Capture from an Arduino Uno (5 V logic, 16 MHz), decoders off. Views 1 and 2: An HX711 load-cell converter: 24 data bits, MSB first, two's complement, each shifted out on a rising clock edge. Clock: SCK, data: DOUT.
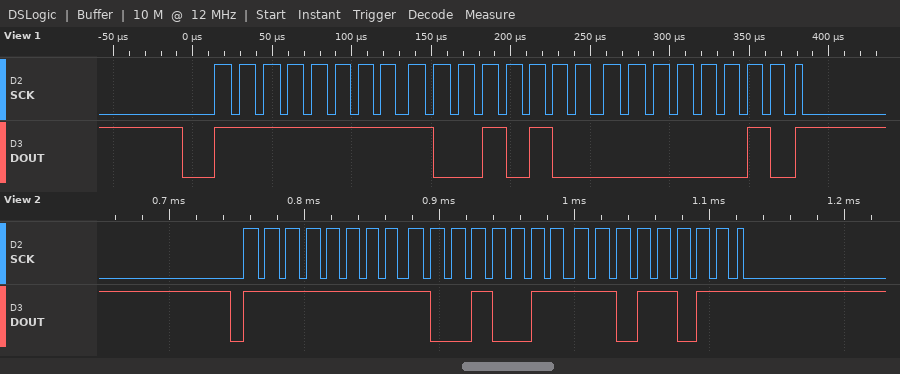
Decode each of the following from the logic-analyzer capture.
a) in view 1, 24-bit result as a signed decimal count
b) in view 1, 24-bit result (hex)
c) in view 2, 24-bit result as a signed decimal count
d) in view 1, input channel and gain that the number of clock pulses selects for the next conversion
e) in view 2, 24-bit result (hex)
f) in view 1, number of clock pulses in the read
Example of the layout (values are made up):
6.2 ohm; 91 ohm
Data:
-27646; 0xFF9402; -27685; channel A, gain 128; 0xFF93DB; 25
